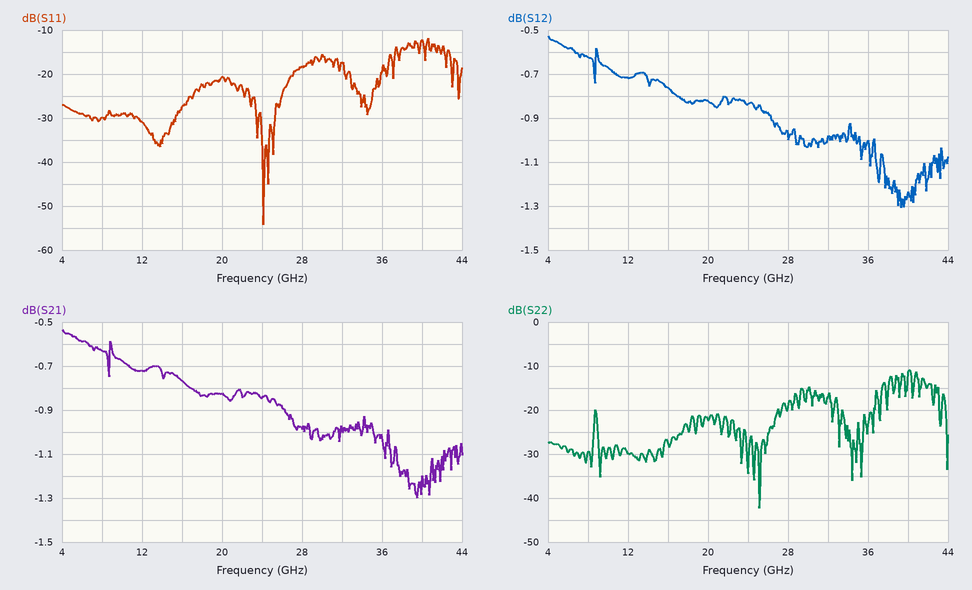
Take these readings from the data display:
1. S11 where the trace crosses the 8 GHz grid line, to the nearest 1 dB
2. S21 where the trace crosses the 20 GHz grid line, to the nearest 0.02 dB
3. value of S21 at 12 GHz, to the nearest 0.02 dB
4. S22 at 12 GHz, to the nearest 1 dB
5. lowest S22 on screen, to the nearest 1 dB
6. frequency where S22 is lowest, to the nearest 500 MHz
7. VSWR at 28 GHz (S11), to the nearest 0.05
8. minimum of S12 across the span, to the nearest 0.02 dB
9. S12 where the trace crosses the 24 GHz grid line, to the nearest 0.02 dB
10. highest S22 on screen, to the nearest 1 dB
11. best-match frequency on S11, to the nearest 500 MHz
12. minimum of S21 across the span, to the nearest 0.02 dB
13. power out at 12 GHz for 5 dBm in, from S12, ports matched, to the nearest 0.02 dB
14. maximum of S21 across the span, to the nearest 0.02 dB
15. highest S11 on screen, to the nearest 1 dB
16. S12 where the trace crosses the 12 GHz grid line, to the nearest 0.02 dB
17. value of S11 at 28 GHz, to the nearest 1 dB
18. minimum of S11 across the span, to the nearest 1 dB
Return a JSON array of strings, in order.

["-30 dB", "-0.82 dB", "-0.72 dB", "-30 dB", "-42 dB", "25.0 GHz", "1.30", "-1.30 dB", "-0.84 dB", "-11 dB", "24.0 GHz", "-1.30 dB", "4.28 dBm", "-0.54 dB", "-12 dB", "-0.72 dB", "-18 dB", "-54 dB"]
